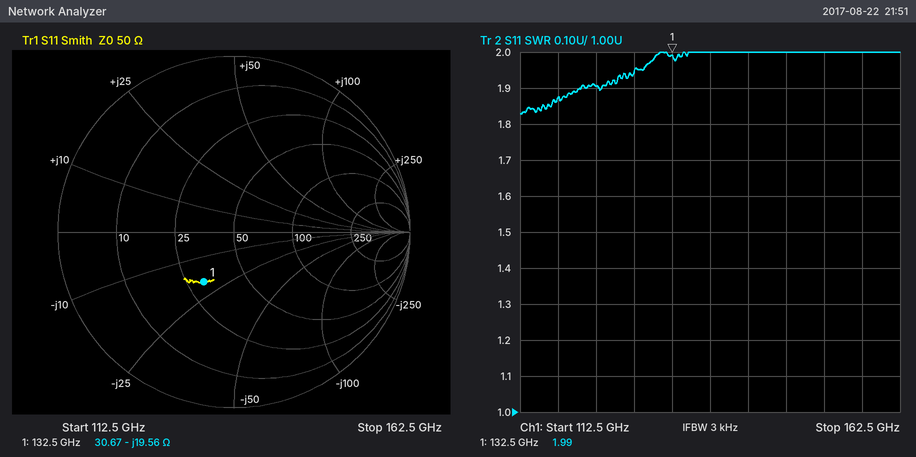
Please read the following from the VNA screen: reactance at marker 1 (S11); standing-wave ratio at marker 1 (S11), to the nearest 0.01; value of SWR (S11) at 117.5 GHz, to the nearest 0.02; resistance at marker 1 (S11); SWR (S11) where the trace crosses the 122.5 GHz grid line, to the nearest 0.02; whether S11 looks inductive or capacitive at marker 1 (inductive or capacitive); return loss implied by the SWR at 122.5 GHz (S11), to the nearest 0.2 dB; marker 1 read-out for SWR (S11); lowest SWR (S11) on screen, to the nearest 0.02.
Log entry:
-19.56 Ω
1.99
1.88
30.67 Ω
1.90
capacitive
10.2 dB
1.99
1.82
